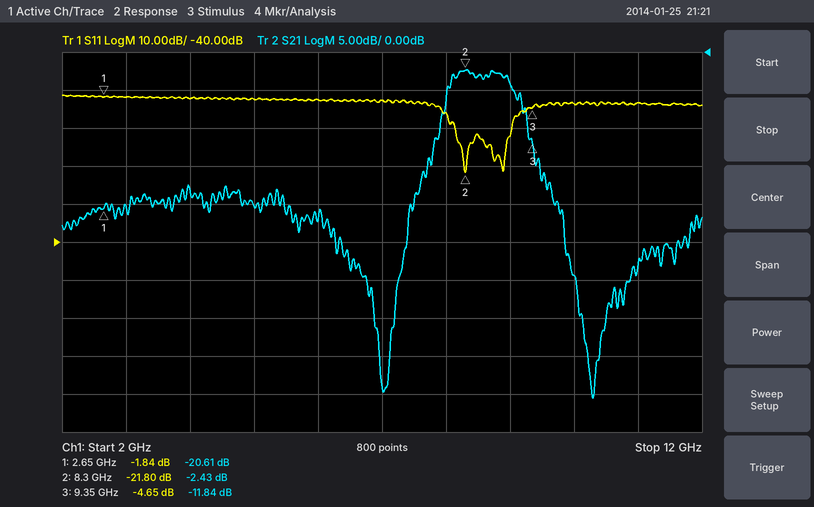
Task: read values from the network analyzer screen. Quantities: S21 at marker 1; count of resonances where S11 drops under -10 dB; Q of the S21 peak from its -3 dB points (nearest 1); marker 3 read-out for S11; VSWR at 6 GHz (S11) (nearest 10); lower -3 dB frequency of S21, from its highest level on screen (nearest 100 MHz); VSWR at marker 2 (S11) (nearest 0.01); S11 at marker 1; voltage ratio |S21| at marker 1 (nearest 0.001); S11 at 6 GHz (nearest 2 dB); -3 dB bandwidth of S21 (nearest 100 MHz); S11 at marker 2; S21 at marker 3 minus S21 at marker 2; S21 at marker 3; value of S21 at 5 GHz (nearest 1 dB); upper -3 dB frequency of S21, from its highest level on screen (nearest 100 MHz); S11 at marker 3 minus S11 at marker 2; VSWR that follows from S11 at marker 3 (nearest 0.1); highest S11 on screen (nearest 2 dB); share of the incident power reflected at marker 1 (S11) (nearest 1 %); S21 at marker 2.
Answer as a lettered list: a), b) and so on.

a) -20.61 dB
b) 2
c) 8
d) -4.65 dB
e) 10
f) 8.0 GHz
g) 1.18
h) -1.84 dB
i) 0.093
j) -2 dB
k) 1.1 GHz
l) -21.80 dB
m) -9.41 dB
n) -11.84 dB
o) -20 dB
p) 9.1 GHz
q) 17.15 dB
r) 3.8
s) -2 dB
t) 65 %
u) -2.43 dB
